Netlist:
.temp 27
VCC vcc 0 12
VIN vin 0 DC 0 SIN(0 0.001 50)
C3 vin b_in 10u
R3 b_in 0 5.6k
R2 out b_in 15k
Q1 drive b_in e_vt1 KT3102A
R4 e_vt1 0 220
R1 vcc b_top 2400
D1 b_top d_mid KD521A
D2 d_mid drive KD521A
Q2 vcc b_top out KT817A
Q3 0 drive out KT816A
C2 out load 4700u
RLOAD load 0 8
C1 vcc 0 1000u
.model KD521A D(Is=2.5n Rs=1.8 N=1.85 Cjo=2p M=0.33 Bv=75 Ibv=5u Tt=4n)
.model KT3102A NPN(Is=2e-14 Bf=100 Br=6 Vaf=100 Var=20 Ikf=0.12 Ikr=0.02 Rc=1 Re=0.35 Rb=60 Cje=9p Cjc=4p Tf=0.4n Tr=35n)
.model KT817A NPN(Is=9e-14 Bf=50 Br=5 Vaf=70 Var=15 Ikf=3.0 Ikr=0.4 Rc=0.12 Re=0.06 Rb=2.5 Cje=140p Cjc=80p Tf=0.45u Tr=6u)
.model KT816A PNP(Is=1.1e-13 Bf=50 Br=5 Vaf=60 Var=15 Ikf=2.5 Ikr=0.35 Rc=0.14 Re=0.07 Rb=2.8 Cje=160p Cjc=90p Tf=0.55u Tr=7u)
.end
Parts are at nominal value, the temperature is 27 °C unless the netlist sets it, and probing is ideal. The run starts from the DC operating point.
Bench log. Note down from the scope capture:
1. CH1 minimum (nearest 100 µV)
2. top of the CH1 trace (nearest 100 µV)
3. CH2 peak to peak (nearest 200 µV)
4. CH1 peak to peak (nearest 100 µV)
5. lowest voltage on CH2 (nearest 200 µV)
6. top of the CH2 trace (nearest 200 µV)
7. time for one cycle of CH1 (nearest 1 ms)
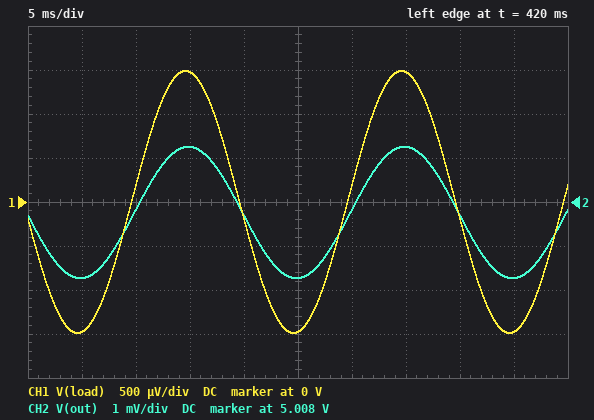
-1.5 mV
1.5 mV
3.0 mV
3.0 mV
5.0062 V
5.0092 V
20 ms
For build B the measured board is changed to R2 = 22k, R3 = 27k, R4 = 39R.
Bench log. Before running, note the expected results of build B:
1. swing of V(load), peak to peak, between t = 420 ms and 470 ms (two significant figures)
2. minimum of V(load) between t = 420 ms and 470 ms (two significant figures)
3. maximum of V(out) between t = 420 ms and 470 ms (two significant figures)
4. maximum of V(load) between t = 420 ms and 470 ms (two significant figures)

14 mV
-7.1 mV
2.4 V
7.1 mV
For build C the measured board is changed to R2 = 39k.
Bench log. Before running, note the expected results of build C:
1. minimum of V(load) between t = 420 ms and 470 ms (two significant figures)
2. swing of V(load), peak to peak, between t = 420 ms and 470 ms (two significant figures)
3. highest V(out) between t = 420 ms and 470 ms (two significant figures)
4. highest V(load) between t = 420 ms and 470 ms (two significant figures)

-1.4 mV
2.8 mV
8.1 V
1.4 mV
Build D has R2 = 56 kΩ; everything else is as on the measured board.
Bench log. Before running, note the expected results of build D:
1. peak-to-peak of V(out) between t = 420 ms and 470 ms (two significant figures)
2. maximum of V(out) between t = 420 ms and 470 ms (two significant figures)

2.5 mV
9.4 V
